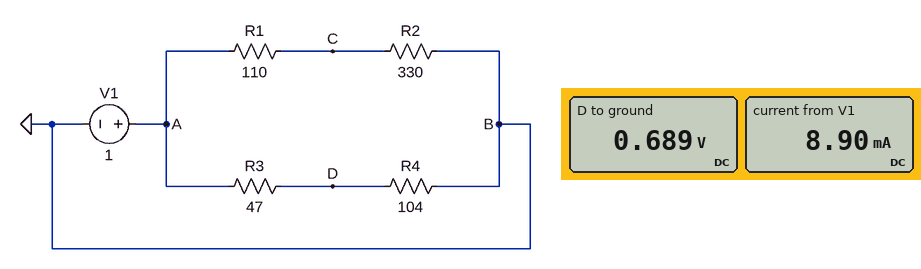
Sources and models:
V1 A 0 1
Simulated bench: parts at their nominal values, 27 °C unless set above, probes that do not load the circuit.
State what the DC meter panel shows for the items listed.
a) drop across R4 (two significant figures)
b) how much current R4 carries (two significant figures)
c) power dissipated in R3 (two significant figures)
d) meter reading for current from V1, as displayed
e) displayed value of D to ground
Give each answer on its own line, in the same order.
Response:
690 mV
6.6 mA
2.1 mW
8.90 mA
0.689 V
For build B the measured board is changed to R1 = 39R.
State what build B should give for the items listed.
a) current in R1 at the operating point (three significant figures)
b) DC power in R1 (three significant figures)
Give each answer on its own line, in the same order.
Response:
2.71 mA
286 µW
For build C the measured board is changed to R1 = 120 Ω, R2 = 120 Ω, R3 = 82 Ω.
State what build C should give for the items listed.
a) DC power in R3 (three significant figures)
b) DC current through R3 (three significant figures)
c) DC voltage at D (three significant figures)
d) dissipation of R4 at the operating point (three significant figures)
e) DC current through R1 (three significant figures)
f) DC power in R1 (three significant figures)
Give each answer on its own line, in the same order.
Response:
2.37 mW
5.38 mA
559 mV
3.01 mW
4.17 mA
2.08 mW
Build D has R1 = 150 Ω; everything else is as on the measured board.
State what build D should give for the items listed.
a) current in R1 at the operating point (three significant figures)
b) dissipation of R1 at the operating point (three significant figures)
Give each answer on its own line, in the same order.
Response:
2.08 mA
651 µW
